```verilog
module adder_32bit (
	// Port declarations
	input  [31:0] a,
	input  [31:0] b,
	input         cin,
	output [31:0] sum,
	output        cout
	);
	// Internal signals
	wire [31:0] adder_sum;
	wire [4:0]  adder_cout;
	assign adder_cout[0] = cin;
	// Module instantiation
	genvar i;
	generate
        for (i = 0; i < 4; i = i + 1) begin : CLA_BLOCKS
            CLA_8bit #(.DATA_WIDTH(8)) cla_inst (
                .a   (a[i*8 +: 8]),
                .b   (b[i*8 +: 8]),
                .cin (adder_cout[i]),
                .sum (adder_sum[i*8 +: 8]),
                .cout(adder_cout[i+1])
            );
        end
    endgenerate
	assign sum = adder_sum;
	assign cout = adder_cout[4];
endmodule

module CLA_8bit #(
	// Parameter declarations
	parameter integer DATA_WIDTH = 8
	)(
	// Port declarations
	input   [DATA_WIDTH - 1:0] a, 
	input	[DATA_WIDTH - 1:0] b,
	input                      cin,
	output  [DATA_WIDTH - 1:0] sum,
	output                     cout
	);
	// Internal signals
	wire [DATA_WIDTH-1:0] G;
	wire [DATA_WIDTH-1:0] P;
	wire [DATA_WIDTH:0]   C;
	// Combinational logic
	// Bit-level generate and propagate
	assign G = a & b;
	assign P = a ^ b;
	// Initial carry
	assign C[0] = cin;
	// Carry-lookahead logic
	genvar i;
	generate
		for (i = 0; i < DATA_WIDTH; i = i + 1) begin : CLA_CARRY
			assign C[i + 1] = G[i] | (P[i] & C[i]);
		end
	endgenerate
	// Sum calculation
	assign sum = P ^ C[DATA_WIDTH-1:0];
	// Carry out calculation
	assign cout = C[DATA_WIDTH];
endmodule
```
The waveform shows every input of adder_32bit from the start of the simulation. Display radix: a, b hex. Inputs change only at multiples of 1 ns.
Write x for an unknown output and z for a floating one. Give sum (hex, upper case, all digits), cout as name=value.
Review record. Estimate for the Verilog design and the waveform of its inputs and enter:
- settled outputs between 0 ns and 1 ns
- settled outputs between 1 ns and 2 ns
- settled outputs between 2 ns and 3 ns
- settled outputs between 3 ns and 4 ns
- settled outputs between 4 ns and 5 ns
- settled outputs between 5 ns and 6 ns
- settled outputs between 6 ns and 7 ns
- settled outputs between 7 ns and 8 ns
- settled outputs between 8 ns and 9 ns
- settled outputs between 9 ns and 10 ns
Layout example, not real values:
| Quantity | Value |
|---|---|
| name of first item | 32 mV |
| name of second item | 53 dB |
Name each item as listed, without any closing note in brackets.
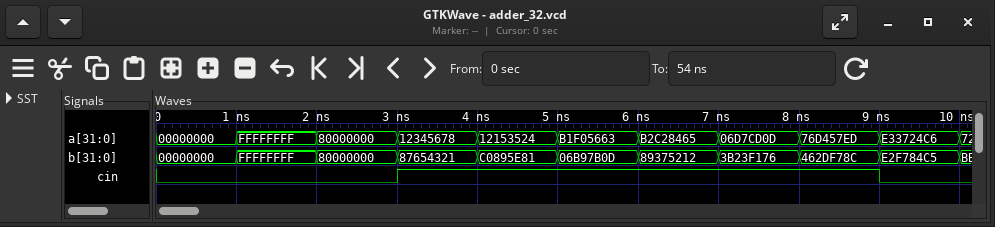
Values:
| Quantity | Value |
|---|---|
| settled outputs between 0 ns and 1 ns | sum=00000000, cout=0 |
| settled outputs between 1 ns and 2 ns | sum=FFFFFFFE, cout=1 |
| settled outputs between 2 ns and 3 ns | sum=00000000, cout=1 |
| settled outputs between 3 ns and 4 ns | sum=9999999A, cout=0 |
| settled outputs between 4 ns and 5 ns | sum=D29E93A6, cout=0 |
| settled outputs between 5 ns and 6 ns | sum=B8A9D171, cout=0 |
| settled outputs between 6 ns and 7 ns | sum=3BF9D678, cout=1 |
| settled outputs between 7 ns and 8 ns | sum=41FBBE84, cout=0 |
| settled outputs between 8 ns and 9 ns | sum=BD024F7A, cout=0 |
| settled outputs between 9 ns and 10 ns | sum=C62EA98B, cout=1 |
